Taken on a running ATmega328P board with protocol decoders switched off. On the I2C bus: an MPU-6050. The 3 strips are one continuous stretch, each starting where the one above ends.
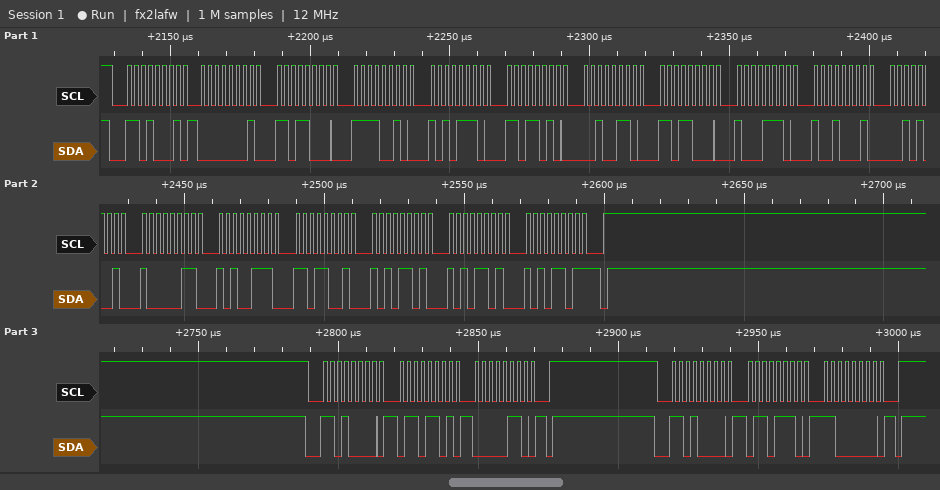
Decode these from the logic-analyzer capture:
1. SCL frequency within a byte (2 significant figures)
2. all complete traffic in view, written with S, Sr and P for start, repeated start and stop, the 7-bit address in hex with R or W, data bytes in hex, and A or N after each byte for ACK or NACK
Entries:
400 kHz
S 68R A 01 A D8 A F2 A AE A DA A 26 A D8 A 8E A 91 A 29 A 83 A A7 A D9 A AD A AD A AD N P S 68W A 6D A 06 A P S 68W A 6E A C0 A P
